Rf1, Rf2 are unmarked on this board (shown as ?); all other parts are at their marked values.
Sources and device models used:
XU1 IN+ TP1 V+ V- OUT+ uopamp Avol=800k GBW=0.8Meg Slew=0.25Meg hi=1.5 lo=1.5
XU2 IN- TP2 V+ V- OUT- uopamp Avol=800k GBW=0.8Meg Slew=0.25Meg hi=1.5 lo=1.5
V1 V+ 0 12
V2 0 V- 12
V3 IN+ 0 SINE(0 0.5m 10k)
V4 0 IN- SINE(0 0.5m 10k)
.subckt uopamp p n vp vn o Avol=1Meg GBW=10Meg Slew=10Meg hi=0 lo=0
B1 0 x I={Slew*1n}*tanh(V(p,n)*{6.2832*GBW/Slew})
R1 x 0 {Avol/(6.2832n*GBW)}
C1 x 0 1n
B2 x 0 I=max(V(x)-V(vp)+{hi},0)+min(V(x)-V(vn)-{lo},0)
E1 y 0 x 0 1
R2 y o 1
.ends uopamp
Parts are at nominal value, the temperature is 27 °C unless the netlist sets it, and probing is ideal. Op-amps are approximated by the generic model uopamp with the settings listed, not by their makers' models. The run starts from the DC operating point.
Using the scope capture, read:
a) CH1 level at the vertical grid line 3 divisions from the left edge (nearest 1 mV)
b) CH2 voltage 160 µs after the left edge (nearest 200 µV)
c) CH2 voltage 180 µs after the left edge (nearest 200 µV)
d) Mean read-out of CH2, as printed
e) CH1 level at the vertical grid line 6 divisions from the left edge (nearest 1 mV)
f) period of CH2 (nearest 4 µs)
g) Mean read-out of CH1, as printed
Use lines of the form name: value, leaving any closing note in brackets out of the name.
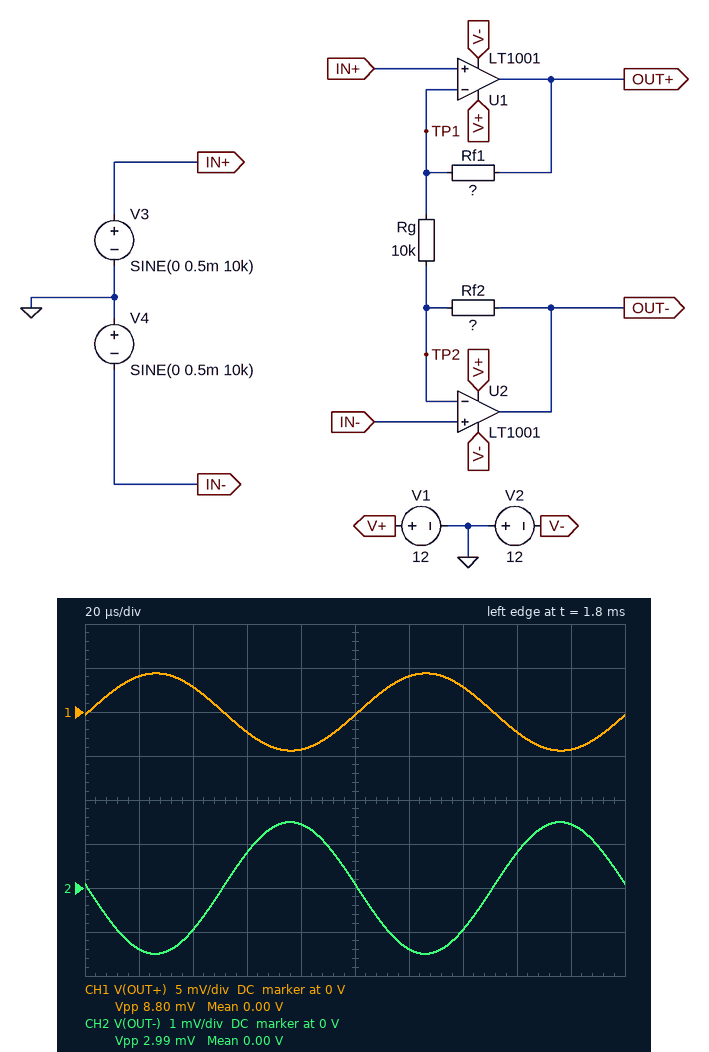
CH1 level at the vertical grid line 3 divisions from the left edge: -2 mV
CH2 voltage 160 µs after the left edge: 800 µV
CH2 voltage 180 µs after the left edge: 1.4 mV
Mean read-out of CH2, as printed: 0.00 V
CH1 level at the vertical grid line 6 divisions from the left edge: 4 mV
period of CH2: 100 µs
Mean read-out of CH1, as printed: 0.00 V
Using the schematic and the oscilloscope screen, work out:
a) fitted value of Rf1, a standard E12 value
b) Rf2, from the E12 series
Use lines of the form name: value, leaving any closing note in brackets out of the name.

fitted value of Rf1, a standard E12 value: 39 kΩ
Rf2, from the E12 series: 10 kΩ
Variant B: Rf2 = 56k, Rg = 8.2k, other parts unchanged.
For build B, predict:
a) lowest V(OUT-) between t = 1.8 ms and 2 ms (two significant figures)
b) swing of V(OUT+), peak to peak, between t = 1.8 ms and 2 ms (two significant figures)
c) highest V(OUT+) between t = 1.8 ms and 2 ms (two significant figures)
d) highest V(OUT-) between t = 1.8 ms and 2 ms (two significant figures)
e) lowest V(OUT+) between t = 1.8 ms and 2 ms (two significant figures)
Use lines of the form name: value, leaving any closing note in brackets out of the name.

lowest V(OUT-) between t = 1.8 ms and 2 ms: -7.2 mV
swing of V(OUT+), peak to peak, between t = 1.8 ms and 2 ms: 10 mV
highest V(OUT+) between t = 1.8 ms and 2 ms: 5.2 mV
highest V(OUT-) between t = 1.8 ms and 2 ms: 7.2 mV
lowest V(OUT+) between t = 1.8 ms and 2 ms: -5.2 mV
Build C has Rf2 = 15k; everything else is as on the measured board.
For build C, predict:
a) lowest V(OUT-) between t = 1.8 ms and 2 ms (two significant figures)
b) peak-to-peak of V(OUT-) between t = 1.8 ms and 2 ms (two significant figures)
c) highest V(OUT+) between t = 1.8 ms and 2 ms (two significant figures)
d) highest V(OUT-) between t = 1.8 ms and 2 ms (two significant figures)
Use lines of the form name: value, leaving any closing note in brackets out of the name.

lowest V(OUT-) between t = 1.8 ms and 2 ms: -2.0 mV
peak-to-peak of V(OUT-) between t = 1.8 ms and 2 ms: 4.0 mV
highest V(OUT+) between t = 1.8 ms and 2 ms: 4.4 mV
highest V(OUT-) between t = 1.8 ms and 2 ms: 2.0 mV
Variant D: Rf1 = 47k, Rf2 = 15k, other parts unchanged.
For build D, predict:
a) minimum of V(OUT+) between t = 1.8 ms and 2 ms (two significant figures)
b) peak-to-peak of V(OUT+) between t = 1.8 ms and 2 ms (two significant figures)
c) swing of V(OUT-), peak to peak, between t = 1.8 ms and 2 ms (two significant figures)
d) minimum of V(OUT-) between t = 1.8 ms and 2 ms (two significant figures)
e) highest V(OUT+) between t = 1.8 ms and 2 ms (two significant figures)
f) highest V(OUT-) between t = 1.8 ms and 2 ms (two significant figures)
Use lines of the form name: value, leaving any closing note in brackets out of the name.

minimum of V(OUT+) between t = 1.8 ms and 2 ms: -5.2 mV
peak-to-peak of V(OUT+) between t = 1.8 ms and 2 ms: 10 mV
swing of V(OUT-), peak to peak, between t = 1.8 ms and 2 ms: 4.0 mV
minimum of V(OUT-) between t = 1.8 ms and 2 ms: -2.0 mV
highest V(OUT+) between t = 1.8 ms and 2 ms: 5.2 mV
highest V(OUT-) between t = 1.8 ms and 2 ms: 2.0 mV
